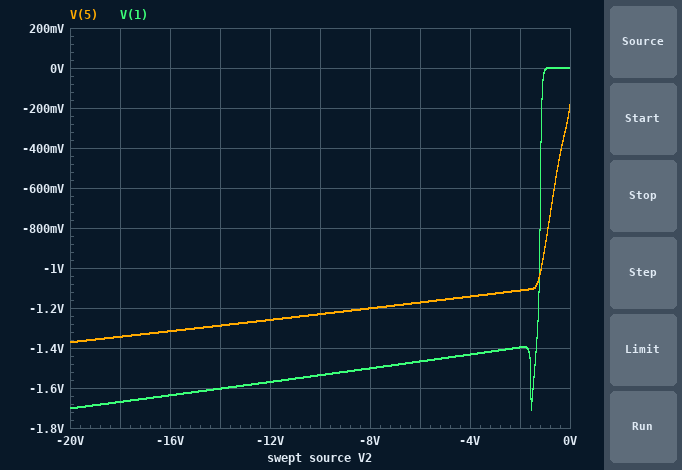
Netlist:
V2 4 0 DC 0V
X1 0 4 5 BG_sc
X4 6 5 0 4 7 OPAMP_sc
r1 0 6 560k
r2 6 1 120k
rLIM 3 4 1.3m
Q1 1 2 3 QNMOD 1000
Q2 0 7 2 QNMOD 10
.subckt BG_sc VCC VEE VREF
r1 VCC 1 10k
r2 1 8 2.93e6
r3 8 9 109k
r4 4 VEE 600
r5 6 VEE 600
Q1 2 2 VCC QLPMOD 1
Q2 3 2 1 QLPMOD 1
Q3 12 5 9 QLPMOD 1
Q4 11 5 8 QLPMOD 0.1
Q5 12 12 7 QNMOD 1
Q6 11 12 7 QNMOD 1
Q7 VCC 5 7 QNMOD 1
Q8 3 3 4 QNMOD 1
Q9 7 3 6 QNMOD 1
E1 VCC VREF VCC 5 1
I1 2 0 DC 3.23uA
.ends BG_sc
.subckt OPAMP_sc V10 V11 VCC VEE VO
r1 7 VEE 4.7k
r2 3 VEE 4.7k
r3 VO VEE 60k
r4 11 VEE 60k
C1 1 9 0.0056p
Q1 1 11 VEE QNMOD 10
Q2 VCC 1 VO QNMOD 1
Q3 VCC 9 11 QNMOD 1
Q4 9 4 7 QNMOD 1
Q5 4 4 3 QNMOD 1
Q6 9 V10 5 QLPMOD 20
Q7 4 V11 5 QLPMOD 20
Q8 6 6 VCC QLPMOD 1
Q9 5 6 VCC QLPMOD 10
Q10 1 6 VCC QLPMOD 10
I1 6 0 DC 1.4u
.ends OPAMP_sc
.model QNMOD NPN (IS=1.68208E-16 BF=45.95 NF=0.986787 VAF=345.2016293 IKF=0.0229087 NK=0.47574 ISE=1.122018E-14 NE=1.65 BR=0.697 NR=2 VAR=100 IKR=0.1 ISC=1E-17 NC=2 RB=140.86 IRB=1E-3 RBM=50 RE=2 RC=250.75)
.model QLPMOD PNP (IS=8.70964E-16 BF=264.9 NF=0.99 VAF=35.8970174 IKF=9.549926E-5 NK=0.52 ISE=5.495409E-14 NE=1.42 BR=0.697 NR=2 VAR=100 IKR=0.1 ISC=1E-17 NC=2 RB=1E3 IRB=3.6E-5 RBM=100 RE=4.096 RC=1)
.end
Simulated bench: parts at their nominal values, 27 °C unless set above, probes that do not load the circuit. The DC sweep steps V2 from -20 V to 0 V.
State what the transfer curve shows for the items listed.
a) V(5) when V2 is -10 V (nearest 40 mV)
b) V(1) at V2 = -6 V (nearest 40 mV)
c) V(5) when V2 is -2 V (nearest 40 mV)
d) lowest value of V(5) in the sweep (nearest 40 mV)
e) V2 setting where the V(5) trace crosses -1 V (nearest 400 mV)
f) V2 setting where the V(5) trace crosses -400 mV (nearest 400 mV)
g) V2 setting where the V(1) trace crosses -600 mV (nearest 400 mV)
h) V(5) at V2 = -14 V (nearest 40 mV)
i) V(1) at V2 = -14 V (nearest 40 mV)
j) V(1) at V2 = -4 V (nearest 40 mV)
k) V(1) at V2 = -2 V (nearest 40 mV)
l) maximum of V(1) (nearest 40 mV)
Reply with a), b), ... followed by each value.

a) -1.24 V
b) -1.48 V
c) -1.12 V
d) -1.36 V
e) -1.2 V
f) -400 mV
g) -1.2 V
h) -1.28 V
i) -1.60 V
j) -1.44 V
k) -1.40 V
l) 0 V
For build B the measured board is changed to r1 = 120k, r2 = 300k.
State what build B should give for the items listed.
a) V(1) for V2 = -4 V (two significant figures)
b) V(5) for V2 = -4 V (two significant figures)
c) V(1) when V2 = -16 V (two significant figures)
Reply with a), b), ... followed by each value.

a) -4.1 V
b) -1.1 V
c) -4.7 V
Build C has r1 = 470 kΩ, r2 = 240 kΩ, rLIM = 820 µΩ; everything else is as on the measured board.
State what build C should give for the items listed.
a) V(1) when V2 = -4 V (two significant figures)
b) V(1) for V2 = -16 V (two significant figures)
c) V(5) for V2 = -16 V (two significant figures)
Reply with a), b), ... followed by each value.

a) -1.8 V
b) -2.1 V
c) -1.3 V
